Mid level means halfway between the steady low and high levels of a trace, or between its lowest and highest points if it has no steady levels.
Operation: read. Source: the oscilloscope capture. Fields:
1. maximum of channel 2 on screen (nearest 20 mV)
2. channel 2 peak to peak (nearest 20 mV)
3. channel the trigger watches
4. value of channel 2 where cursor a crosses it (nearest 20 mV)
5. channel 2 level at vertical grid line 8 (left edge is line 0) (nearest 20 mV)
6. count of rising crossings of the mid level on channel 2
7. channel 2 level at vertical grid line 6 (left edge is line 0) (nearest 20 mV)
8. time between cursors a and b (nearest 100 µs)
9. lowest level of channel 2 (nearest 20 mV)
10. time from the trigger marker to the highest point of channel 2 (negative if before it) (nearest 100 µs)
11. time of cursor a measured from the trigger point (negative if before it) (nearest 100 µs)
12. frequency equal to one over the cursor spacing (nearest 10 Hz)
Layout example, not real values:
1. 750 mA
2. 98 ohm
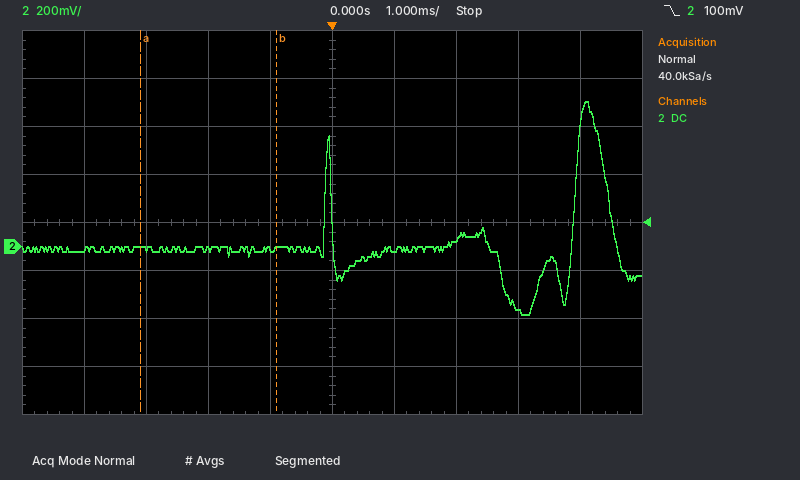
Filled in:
1. 600 mV
2. 880 mV
3. channel 2
4. 0 mV
5. -260 mV
6. 2
7. -20 mV
8. 2.2 ms
9. -280 mV
10. +4.1 ms
11. -3.1 ms
12. 450 Hz
